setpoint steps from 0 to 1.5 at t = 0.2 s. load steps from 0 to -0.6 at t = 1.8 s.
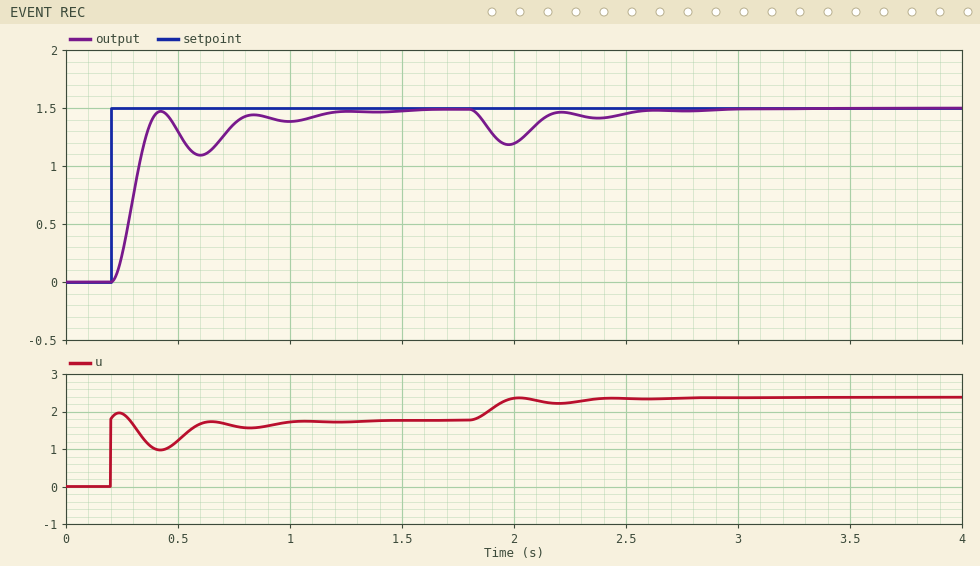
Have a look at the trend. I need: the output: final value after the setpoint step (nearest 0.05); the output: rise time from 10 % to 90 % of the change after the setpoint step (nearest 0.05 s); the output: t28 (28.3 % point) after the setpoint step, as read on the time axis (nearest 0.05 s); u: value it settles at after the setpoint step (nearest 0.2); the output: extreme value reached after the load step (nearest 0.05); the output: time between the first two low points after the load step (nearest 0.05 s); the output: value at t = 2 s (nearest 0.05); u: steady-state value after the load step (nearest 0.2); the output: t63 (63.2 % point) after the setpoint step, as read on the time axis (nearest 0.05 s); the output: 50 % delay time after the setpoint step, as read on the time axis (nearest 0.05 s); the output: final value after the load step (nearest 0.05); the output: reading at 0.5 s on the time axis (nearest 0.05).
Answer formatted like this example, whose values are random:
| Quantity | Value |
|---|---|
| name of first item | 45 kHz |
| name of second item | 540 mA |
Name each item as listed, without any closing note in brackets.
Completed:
| Quantity | Value |
|---|---|
| the output: final value after the setpoint step | 1.50 |
| the output: rise time from 10 % to 90 % of the change after the setpoint step | 0.15 s |
| the output: t28 (28.3 % point) after the setpoint step, as read on the time axis | 0.25 s |
| u: value it settles at after the setpoint step | 1.8 |
| the output: extreme value reached after the load step | 1.20 |
| the output: time between the first two low points after the load step | 0.40 s |
| the output: value at t = 2 s | 1.20 |
| u: steady-state value after the load step | 2.4 |
| the output: t63 (63.2 % point) after the setpoint step, as read on the time axis | 0.30 s |
| the output: 50 % delay time after the setpoint step, as read on the time axis | 0.30 s |
| the output: final value after the load step | 1.50 |
| the output: reading at 0.5 s on the time axis | 1.30 |
